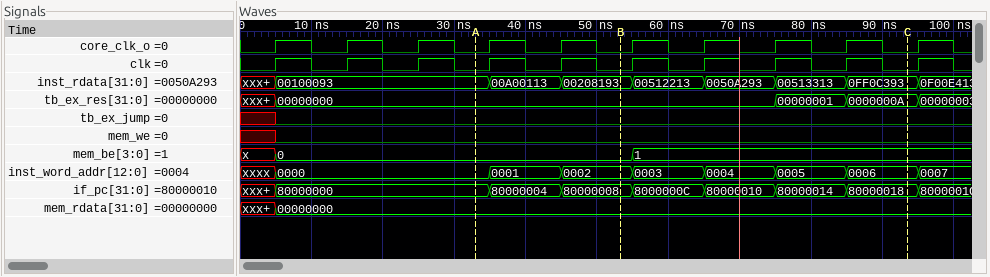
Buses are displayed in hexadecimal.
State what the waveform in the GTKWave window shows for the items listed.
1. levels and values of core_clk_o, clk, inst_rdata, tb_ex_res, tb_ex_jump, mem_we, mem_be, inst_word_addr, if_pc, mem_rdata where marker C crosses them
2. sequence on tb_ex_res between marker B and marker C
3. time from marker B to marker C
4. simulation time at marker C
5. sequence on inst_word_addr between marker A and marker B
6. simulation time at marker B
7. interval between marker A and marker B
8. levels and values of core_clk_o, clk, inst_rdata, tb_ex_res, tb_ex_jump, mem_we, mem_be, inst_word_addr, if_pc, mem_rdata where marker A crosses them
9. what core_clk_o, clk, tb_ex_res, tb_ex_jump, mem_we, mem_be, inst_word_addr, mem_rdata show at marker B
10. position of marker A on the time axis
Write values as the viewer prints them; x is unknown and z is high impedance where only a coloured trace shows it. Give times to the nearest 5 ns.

core_clk_o=0, clk=0, inst_rdata=0FF0C393, tb_ex_res=0000000A, tb_ex_jump=0, mem_we=0, mem_be=1, inst_word_addr=0006, if_pc=80000018, mem_rdata=00000000
00000000, 00000001, 0000000A
40 ns
95 ns
0000, 0001, 0002
55 ns
20 ns
core_clk_o=0, clk=0, inst_rdata=00100093, tb_ex_res=00000000, tb_ex_jump=0, mem_we=0, mem_be=0, inst_word_addr=0000, if_pc=80000000, mem_rdata=00000000
core_clk_o=0, clk=0, tb_ex_res=00000000, tb_ex_jump=0, mem_we=0, mem_be=0, inst_word_addr=0002, mem_rdata=00000000
35 ns
